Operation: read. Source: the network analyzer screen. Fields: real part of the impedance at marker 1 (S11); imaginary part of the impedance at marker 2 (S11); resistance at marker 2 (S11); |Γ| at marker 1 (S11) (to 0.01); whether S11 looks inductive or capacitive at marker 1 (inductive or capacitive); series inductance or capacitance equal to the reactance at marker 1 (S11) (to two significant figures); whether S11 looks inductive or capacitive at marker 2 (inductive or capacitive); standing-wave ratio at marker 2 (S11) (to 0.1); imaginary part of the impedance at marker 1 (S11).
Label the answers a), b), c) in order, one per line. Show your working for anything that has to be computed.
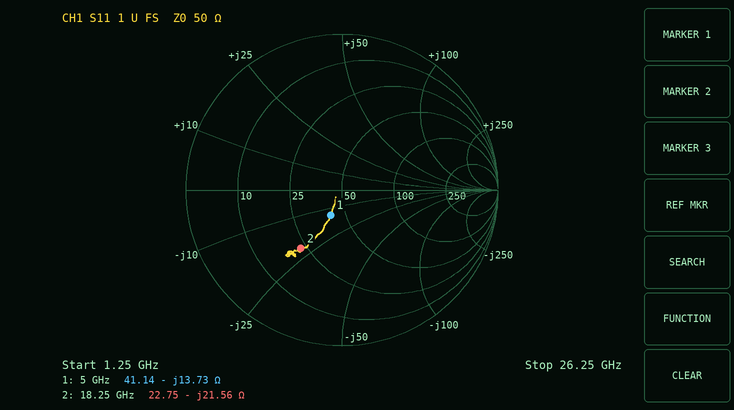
a) 41.14 Ω
b) -21.56 Ω
c) 22.75 Ω
d) 0.18
e) capacitive
f) C = 1/(2π × 5 GHz × 13.73 Ω) ≈ 2.3 pF
g) capacitive
h) 2.7
i) -13.73 Ω
